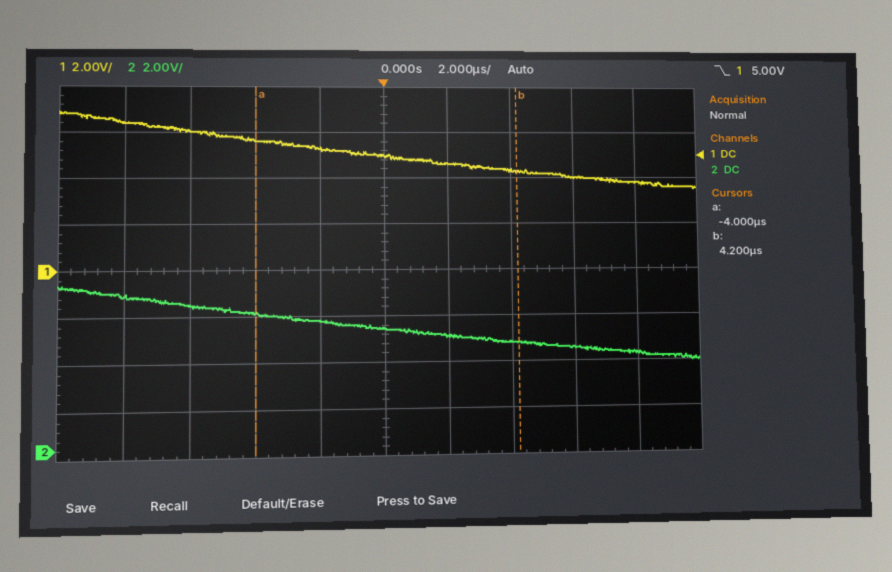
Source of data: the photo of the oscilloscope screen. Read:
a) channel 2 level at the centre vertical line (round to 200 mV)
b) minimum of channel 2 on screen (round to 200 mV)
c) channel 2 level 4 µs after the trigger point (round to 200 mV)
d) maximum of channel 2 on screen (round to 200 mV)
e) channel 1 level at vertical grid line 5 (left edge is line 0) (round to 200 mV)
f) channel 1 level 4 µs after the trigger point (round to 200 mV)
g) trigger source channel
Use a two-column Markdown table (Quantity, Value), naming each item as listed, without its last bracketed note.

| Quantity | Value |
|---|---|
| channel 2 level at the centre vertical line | 5.0 V |
| minimum of channel 2 on screen | 3.6 V |
| channel 2 level 4 µs after the trigger point | 4.4 V |
| maximum of channel 2 on screen | 7.0 V |
| channel 1 level at vertical grid line 5 (left edge is line 0) | 5.0 V |
| channel 1 level 4 µs after the trigger point | 4.4 V |
| trigger source channel | channel 1 |
